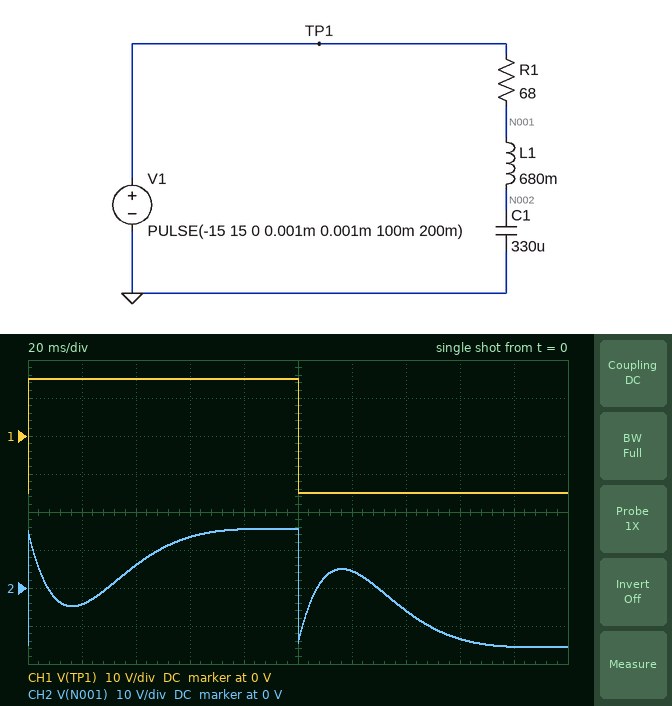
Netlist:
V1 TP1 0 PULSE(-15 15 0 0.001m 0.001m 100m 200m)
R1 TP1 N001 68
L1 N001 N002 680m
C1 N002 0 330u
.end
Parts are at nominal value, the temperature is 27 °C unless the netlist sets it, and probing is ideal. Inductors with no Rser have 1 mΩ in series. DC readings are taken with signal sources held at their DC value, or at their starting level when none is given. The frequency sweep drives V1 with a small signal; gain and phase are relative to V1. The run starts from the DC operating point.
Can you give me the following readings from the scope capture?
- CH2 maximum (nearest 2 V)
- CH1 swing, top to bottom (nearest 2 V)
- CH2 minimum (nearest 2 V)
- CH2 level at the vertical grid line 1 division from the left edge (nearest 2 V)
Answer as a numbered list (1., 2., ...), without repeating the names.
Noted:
1. 16 V
2. 30 V
3. -16 V
4. -4 V
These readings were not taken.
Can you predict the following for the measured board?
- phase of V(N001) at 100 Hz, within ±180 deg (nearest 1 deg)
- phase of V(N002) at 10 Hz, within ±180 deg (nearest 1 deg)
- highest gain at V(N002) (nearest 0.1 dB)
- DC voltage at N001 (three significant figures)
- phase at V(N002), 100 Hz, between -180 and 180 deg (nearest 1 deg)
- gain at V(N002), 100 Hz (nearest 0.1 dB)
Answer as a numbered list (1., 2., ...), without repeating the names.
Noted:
1. 9 deg
2. -85 deg
3. 0 dB
4. -15.0 V
5. -171 deg
6. -39.0 dB
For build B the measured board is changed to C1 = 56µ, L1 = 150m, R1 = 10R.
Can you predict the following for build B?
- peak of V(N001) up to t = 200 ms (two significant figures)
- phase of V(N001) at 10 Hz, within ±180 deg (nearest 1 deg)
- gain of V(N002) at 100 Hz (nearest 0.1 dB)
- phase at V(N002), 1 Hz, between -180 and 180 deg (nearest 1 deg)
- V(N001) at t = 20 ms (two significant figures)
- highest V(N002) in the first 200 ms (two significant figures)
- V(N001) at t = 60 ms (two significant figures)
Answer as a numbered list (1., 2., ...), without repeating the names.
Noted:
1. 19 V
2. -2 deg
3. -7.4 dB
4. 0 deg
5. 13 V
6. 37 V
7. 14 V
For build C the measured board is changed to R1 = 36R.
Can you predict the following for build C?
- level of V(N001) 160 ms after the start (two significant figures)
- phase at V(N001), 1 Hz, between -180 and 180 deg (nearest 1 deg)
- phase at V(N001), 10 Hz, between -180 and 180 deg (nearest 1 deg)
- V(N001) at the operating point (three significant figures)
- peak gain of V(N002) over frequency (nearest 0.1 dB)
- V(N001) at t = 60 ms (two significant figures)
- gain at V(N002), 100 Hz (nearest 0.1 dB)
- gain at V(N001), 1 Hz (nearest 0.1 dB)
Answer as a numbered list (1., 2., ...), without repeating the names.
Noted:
1. -18 V
2. -4 deg
3. -81 deg
4. -15.0 V
5. 2.8 dB
6. 18 V
7. -38.9 dB
8. 0 dB
